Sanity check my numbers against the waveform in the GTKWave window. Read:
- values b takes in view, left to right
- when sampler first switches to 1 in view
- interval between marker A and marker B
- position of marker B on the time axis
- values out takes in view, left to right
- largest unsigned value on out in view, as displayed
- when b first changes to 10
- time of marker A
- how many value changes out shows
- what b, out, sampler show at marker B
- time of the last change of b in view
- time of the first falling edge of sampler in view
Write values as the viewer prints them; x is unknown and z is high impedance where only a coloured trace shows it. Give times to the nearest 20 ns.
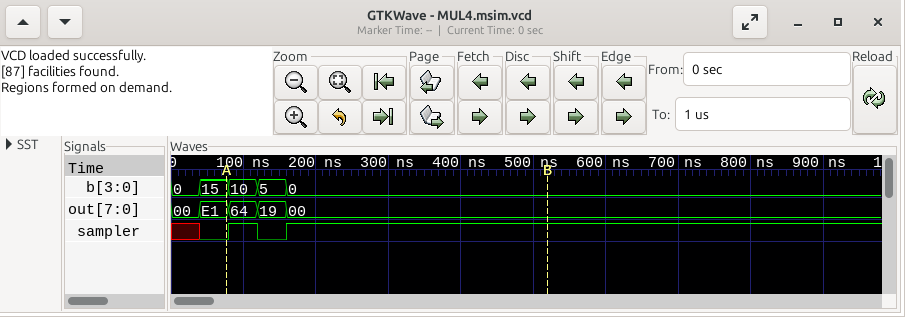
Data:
0, 15, 10, 5, 0
80 ns
440 ns
520 ns
00, E1, 64, 19, 00
E1
80 ns
80 ns
4
b=0, out=00, sampler=1
160 ns
120 ns
